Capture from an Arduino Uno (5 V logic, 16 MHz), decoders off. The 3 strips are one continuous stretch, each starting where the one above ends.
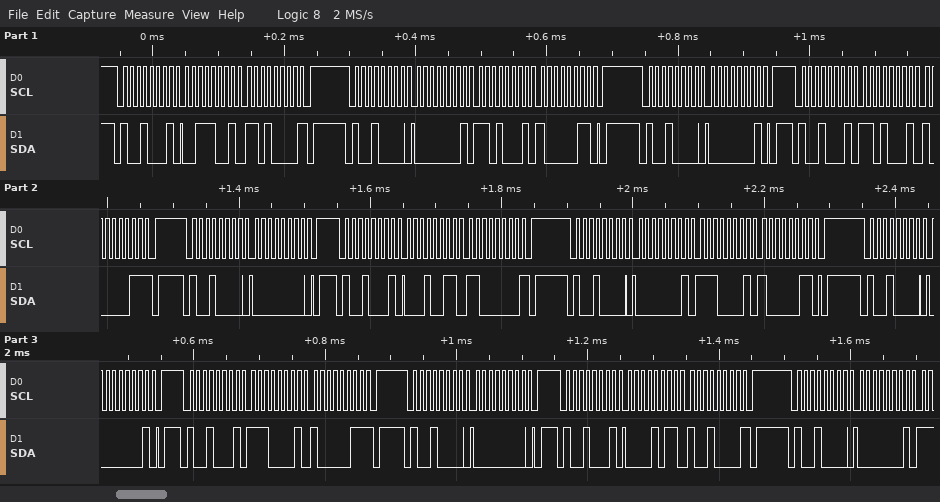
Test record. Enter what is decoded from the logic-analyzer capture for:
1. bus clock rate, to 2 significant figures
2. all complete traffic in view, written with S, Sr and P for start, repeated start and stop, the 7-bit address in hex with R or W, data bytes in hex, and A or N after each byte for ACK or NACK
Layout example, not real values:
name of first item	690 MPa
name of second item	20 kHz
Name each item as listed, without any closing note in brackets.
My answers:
bus clock rate, to 2 significant figures	100 kHz
all complete traffic in view, written with S, Sr and P for start, repeated start and stop, the 7-bit address in hex with R or W, data bytes in hex, and A or N after each byte for ACK or NACK	S 48R A 39 A D0 N P S 48W A 01 A D1 A 83 A P S 48W A 01 A P S 48R A D1 A 83 N P S 48W A 00 A P S 48R A 13 A C0 N P S 48W A 01 A E1 A 83 A P S 48W A 01 A P S 48R A E1 A 83 N P S 48W A 00 A P S 48R A 0B A 90 N P S 48W A 01 A
